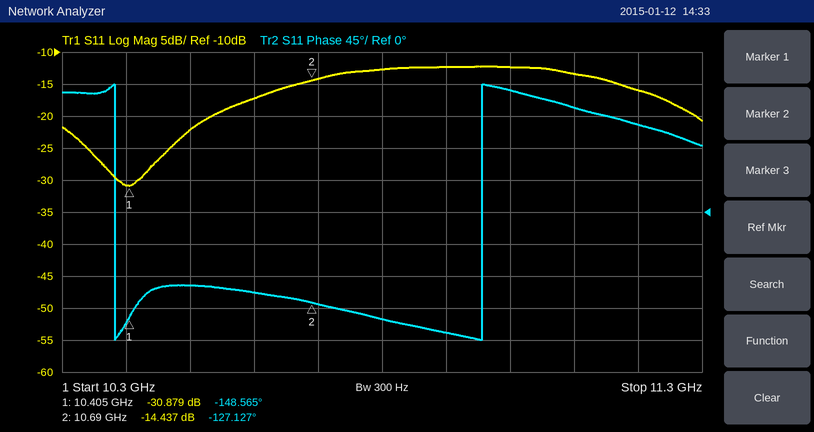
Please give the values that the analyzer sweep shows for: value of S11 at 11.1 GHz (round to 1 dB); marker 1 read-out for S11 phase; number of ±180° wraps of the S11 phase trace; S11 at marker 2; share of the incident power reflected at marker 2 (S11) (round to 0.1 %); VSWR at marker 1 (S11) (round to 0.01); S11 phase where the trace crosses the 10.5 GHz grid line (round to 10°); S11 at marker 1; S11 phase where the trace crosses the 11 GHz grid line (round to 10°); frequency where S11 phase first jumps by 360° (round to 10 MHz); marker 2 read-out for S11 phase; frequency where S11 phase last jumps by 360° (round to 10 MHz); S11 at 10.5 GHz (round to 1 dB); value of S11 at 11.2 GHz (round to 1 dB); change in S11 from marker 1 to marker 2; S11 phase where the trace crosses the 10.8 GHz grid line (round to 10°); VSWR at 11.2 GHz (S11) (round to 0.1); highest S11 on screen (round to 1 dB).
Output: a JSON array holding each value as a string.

["-13 dB", "-148.565°", "2", "-14.437 dB", "3.6 %", "1.06", "-100°", "-30.879 dB", "170°", "10.38 GHz", "-127.127°", "10.96 GHz", "-22 dB", "-16 dB", "16.442 dB", "-150°", "1.4", "-12 dB"]
